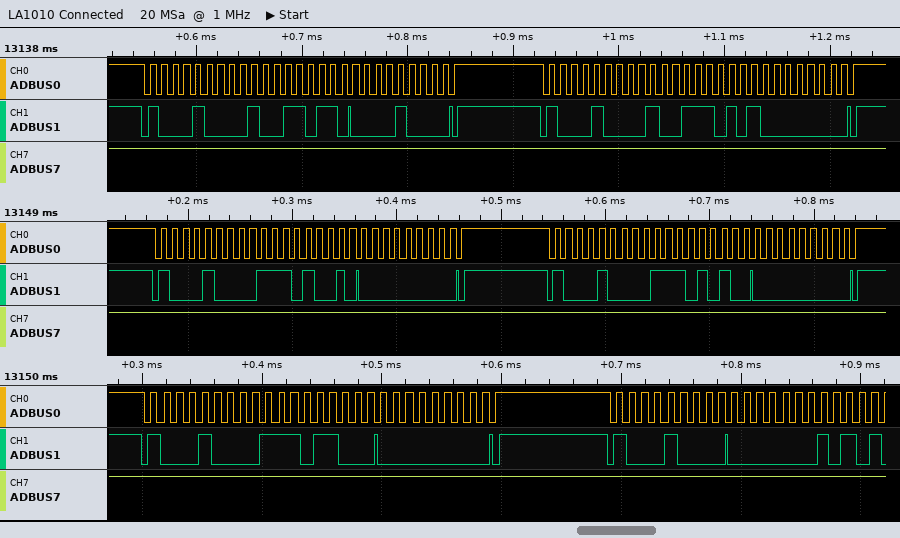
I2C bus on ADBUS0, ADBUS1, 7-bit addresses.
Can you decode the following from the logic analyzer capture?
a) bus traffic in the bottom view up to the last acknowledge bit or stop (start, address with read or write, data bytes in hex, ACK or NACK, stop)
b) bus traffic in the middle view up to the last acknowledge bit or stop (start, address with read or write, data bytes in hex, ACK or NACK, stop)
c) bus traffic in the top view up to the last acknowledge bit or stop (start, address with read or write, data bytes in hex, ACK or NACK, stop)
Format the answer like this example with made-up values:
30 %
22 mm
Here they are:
start, address 44 write ACK, EC ACK, 00 ACK, stop, start, address 44 write ACK, 01 ACK
start, address 44 write ACK, E9 ACK, 00 ACK, stop, start, address 44 write ACK, EA ACK, 00 ACK, stop
start, address 44 write ACK, 9B ACK, 08 ACK, stop, start, address 44 write ACK, 9D ACK, 80 ACK, stop
